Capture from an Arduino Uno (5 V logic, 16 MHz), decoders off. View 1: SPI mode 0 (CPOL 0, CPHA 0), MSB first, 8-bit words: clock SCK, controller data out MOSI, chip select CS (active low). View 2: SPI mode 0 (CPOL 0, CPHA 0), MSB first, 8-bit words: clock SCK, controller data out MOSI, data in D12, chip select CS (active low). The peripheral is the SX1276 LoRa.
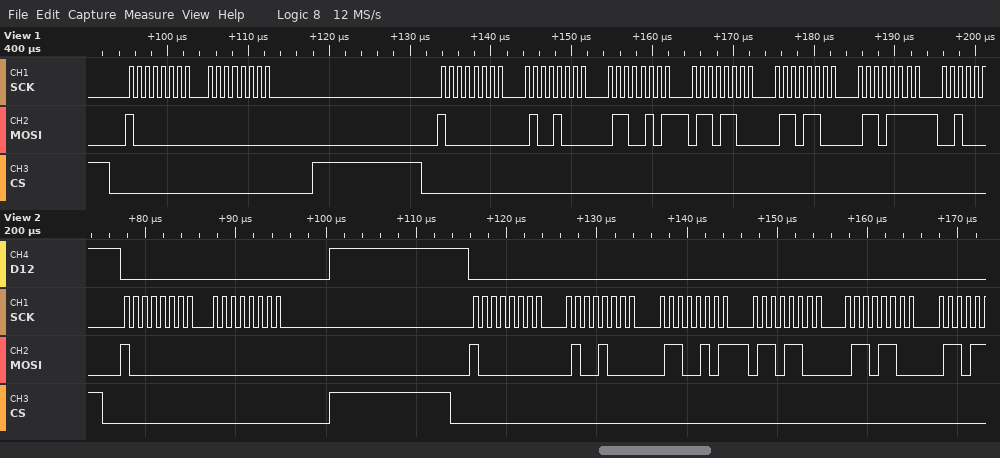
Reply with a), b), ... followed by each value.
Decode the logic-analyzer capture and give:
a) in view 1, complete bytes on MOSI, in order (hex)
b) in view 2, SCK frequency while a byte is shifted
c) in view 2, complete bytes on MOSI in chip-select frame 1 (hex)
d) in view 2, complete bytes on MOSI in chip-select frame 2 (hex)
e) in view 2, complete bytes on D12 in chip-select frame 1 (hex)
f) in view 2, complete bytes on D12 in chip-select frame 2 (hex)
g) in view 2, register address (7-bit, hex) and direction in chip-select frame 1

a) 80 00 80 48 65 6C 6C 6F
b) 1 MHz
c) 0x80 0x00
d) 0x80 0x48 0x65 0x6C 0x6C
e) 0x00 0x00
f) 0x00 0x00 0x00 0x00 0x00
g) 0x00 write
